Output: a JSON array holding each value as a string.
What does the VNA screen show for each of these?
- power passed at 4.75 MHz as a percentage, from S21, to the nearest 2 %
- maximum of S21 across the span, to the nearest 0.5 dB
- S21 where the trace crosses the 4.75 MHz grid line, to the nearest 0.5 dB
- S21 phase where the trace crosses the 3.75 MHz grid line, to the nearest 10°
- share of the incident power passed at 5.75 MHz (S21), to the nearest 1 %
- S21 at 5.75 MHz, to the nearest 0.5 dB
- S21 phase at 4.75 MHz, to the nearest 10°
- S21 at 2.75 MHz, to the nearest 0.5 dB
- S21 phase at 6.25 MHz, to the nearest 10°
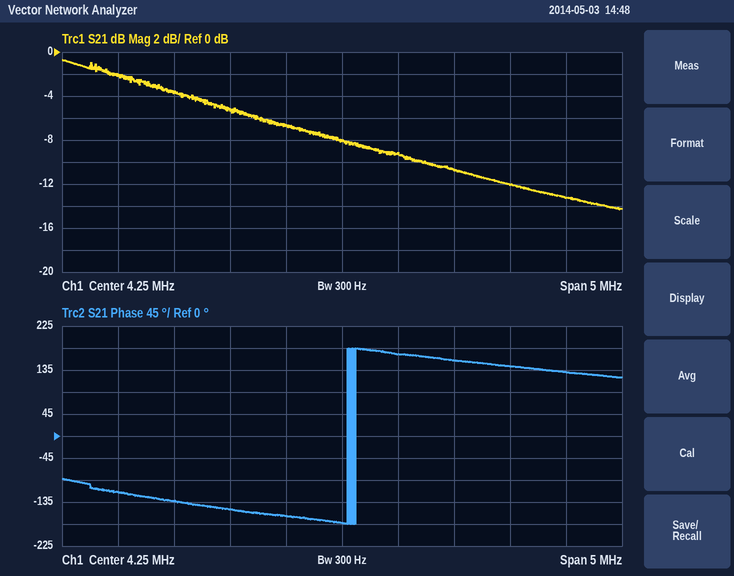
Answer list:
["12 %", "-0.5 dB", "-9.0 dB", "-160°", "6 %", "-12.0 dB", "170°", "-3.5 dB", "130°"]
